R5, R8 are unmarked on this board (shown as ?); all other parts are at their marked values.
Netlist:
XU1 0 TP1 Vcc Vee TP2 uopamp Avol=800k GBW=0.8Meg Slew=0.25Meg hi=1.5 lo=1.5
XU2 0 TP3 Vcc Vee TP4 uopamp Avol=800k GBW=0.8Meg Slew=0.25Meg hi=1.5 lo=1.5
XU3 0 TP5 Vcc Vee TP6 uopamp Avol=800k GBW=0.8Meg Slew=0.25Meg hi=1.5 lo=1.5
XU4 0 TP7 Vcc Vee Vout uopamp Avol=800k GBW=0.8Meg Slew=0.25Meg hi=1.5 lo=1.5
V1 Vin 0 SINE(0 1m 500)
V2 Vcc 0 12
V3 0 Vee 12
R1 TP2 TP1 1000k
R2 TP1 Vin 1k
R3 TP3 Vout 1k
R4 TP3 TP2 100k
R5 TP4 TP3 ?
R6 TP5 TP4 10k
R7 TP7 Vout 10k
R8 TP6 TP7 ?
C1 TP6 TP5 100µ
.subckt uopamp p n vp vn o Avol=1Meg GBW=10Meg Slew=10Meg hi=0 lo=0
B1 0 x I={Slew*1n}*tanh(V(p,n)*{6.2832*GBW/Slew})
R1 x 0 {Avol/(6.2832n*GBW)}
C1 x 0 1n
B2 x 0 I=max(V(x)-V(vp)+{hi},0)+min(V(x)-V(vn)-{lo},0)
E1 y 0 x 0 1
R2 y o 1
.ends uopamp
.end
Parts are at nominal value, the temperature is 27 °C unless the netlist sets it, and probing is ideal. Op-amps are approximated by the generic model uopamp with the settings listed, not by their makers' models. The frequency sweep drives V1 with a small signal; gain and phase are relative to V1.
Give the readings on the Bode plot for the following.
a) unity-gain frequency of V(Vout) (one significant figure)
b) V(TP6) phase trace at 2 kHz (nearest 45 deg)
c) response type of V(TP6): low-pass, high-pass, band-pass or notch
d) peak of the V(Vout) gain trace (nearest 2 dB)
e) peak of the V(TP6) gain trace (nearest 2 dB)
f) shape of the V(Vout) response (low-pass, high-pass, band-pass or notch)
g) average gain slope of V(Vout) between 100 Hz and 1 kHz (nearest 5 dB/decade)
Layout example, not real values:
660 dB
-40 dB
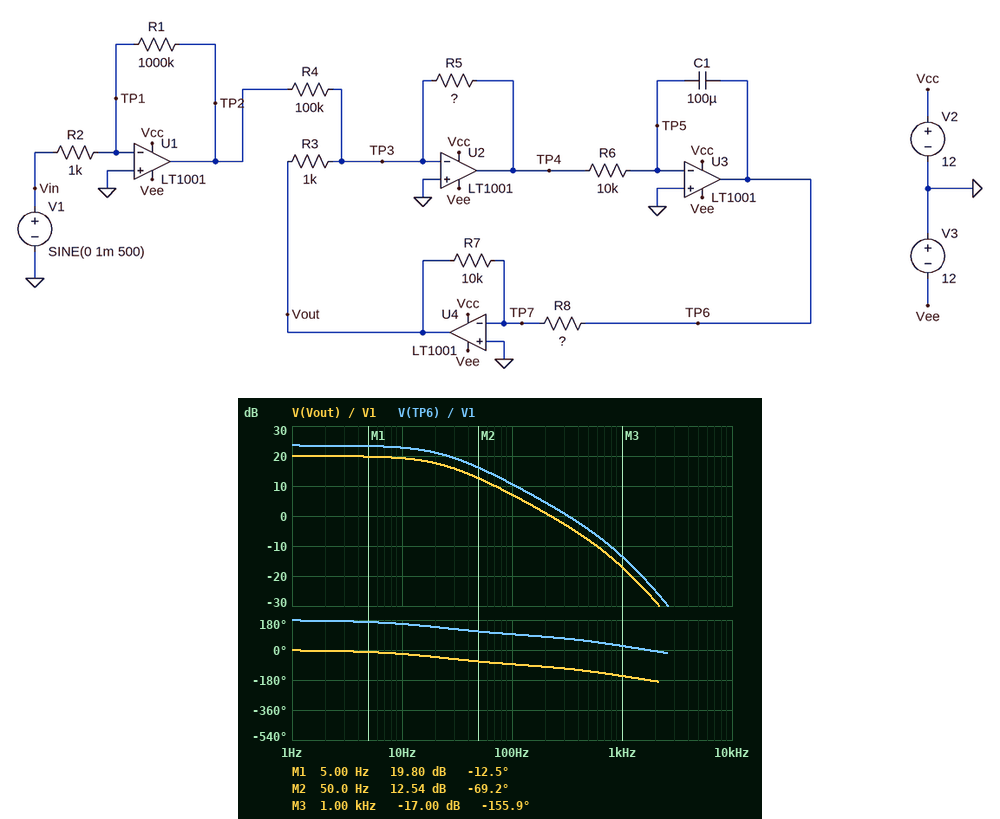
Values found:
200 Hz
0 deg
low-pass
20 dB
24 dB
low-pass
-25 dB/decade
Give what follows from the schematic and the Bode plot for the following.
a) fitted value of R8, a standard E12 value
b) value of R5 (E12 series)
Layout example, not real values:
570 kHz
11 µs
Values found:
15 kΩ
220 kΩ
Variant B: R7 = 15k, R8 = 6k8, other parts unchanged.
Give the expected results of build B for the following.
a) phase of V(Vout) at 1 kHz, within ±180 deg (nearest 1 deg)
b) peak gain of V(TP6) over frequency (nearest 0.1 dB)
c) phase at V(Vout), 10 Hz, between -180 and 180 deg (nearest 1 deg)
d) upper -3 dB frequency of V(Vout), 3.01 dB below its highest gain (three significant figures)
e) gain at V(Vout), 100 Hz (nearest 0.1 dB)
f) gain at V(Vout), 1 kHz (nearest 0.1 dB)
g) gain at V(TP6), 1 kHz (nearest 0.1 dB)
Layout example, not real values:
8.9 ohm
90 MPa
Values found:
-153 deg
13.1 dB
-8 deg
78.2 Hz
15.8 dB
-6.5 dB
-13.4 dB
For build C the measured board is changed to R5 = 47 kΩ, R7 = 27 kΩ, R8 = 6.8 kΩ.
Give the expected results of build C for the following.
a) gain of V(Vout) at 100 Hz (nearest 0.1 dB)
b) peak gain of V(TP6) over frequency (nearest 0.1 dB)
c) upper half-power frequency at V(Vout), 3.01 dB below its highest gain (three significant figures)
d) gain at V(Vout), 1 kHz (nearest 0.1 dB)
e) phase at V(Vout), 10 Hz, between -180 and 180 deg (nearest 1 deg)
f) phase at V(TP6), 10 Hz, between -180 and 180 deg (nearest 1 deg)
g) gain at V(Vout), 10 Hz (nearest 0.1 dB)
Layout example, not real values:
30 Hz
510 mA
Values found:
9.0 dB
8.0 dB
29.7 Hz
-14.6 dB
-19 deg
161 deg
19.5 dB
